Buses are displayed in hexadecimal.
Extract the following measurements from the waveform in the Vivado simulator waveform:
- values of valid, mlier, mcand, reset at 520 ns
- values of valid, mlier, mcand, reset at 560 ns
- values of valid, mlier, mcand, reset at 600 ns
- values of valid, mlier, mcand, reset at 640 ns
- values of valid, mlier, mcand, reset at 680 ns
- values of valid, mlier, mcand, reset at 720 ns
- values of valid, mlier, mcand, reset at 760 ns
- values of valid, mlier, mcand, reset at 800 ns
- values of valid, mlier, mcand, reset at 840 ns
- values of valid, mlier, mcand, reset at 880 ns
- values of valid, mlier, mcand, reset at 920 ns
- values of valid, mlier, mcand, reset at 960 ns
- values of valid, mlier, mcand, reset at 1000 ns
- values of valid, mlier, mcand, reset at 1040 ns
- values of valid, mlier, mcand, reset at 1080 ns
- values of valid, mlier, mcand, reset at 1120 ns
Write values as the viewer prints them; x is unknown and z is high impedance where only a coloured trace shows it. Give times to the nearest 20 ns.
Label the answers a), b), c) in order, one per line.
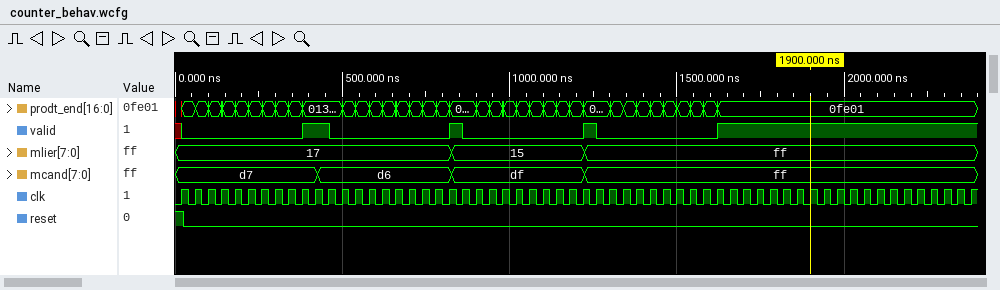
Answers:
a) valid=0, mlier=17, mcand=d6, reset=0
b) valid=0, mlier=17, mcand=d6, reset=0
c) valid=0, mlier=17, mcand=d6, reset=0
d) valid=0, mlier=17, mcand=d6, reset=0
e) valid=0, mlier=17, mcand=d6, reset=0
f) valid=0, mlier=17, mcand=d6, reset=0
g) valid=0, mlier=17, mcand=d6, reset=0
h) valid=0, mlier=17, mcand=d6, reset=0
i) valid=1, mlier=15, mcand=df, reset=0
j) valid=0, mlier=15, mcand=df, reset=0
k) valid=0, mlier=15, mcand=df, reset=0
l) valid=0, mlier=15, mcand=df, reset=0
m) valid=0, mlier=15, mcand=df, reset=0
n) valid=0, mlier=15, mcand=df, reset=0
o) valid=0, mlier=15, mcand=df, reset=0
p) valid=0, mlier=15, mcand=df, reset=0
